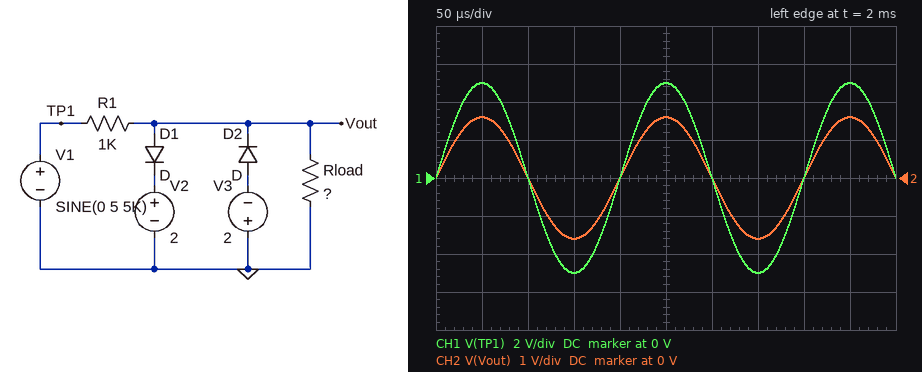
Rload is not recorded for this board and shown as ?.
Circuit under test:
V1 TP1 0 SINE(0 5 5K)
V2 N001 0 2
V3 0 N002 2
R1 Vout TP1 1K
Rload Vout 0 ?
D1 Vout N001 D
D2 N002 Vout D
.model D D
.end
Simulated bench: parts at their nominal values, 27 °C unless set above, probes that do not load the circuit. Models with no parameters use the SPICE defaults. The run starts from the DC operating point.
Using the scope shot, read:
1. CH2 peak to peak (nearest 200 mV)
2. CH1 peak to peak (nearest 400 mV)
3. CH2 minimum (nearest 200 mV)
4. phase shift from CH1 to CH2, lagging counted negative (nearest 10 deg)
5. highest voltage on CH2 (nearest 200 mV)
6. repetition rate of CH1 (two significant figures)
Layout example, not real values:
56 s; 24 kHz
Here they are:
3.2 V; 10.0 V; -1.6 V; 0 deg; 1.6 V; 5.0 kHz
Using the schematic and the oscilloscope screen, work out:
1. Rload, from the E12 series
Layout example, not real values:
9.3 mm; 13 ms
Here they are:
470 Ω
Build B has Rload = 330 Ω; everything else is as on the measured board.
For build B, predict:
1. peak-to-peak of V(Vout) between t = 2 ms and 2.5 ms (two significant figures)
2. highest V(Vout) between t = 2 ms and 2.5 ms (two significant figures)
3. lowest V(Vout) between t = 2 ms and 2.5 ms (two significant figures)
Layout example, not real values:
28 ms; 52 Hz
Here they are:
2.5 V; 1.2 V; -1.2 V
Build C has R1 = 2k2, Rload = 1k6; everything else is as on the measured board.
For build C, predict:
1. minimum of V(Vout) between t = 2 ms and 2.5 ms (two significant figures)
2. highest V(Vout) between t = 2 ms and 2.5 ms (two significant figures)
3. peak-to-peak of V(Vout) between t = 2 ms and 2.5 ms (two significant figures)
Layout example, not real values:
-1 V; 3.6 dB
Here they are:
-2.1 V; 2.1 V; 4.2 V
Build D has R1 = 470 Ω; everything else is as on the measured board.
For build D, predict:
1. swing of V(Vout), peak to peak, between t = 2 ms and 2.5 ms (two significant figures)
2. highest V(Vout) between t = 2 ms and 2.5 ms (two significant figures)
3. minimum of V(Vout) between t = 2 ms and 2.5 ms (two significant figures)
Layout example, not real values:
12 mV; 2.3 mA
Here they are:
5.0 V; 2.5 V; -2.5 V
